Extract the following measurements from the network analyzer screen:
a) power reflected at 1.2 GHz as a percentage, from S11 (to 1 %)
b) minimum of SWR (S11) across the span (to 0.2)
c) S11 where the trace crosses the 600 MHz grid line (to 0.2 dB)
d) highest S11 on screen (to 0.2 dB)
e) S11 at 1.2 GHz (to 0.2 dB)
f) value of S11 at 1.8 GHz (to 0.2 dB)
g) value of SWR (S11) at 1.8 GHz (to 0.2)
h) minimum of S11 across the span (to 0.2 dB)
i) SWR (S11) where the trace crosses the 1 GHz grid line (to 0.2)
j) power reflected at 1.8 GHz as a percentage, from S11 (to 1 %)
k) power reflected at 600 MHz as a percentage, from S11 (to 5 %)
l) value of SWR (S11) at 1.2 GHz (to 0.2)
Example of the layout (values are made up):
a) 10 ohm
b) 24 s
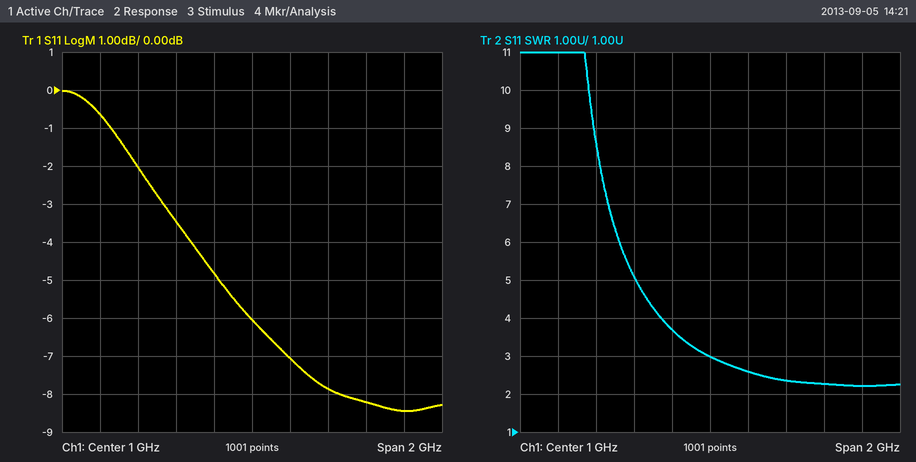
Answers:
a) 20 %
b) 2.2
c) -3.4 dB
d) 0.0 dB
e) -7.0 dB
f) -8.4 dB
g) 2.2
h) -8.4 dB
i) 3.0
j) 14 %
k) 45 %
l) 2.6
